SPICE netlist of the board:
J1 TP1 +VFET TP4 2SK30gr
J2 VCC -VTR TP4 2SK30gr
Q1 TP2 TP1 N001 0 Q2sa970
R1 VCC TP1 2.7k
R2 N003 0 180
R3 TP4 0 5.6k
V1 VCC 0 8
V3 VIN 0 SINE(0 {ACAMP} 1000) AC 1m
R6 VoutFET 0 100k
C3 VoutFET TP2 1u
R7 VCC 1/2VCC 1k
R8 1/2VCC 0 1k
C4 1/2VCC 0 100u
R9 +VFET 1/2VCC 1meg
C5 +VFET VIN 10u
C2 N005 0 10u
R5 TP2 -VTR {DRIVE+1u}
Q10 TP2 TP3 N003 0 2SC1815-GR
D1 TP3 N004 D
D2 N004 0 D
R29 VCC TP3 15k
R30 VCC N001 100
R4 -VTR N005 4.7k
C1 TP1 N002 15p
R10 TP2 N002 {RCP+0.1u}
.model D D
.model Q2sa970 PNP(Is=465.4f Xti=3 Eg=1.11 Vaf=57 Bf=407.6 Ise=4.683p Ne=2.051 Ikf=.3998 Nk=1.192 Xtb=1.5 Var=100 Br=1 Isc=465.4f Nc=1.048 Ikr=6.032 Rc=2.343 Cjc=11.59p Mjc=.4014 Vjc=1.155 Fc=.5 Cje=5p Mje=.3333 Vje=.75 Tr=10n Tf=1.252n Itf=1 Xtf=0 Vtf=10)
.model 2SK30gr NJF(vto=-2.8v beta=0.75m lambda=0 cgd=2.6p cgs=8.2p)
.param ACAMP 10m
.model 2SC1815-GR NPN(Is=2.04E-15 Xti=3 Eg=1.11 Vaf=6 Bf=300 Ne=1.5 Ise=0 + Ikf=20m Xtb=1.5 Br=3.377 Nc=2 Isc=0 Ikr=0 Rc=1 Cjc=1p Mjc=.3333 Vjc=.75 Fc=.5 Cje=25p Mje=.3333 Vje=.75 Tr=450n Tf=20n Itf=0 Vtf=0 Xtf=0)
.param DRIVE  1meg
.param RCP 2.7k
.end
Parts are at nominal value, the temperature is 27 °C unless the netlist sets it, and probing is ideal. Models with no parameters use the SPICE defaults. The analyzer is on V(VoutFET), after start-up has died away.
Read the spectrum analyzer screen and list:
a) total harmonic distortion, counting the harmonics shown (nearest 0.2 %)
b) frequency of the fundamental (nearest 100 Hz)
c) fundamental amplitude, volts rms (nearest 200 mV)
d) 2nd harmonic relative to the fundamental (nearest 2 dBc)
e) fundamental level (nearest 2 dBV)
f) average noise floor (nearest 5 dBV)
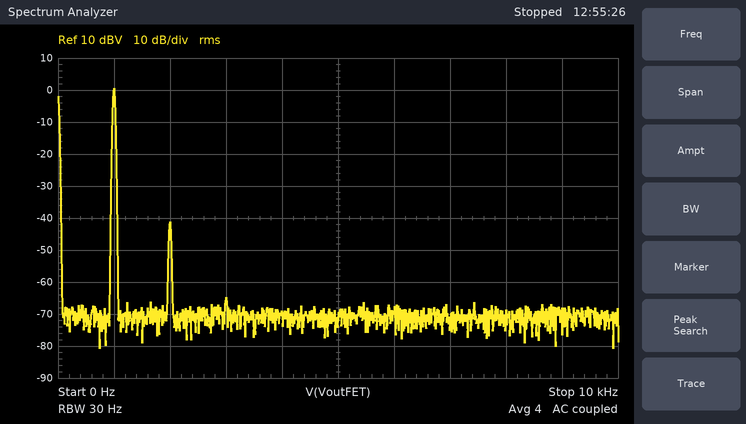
0.8 %
1.0 kHz
1.0 V
-42 dBc
0 dBV
-70 dBV
